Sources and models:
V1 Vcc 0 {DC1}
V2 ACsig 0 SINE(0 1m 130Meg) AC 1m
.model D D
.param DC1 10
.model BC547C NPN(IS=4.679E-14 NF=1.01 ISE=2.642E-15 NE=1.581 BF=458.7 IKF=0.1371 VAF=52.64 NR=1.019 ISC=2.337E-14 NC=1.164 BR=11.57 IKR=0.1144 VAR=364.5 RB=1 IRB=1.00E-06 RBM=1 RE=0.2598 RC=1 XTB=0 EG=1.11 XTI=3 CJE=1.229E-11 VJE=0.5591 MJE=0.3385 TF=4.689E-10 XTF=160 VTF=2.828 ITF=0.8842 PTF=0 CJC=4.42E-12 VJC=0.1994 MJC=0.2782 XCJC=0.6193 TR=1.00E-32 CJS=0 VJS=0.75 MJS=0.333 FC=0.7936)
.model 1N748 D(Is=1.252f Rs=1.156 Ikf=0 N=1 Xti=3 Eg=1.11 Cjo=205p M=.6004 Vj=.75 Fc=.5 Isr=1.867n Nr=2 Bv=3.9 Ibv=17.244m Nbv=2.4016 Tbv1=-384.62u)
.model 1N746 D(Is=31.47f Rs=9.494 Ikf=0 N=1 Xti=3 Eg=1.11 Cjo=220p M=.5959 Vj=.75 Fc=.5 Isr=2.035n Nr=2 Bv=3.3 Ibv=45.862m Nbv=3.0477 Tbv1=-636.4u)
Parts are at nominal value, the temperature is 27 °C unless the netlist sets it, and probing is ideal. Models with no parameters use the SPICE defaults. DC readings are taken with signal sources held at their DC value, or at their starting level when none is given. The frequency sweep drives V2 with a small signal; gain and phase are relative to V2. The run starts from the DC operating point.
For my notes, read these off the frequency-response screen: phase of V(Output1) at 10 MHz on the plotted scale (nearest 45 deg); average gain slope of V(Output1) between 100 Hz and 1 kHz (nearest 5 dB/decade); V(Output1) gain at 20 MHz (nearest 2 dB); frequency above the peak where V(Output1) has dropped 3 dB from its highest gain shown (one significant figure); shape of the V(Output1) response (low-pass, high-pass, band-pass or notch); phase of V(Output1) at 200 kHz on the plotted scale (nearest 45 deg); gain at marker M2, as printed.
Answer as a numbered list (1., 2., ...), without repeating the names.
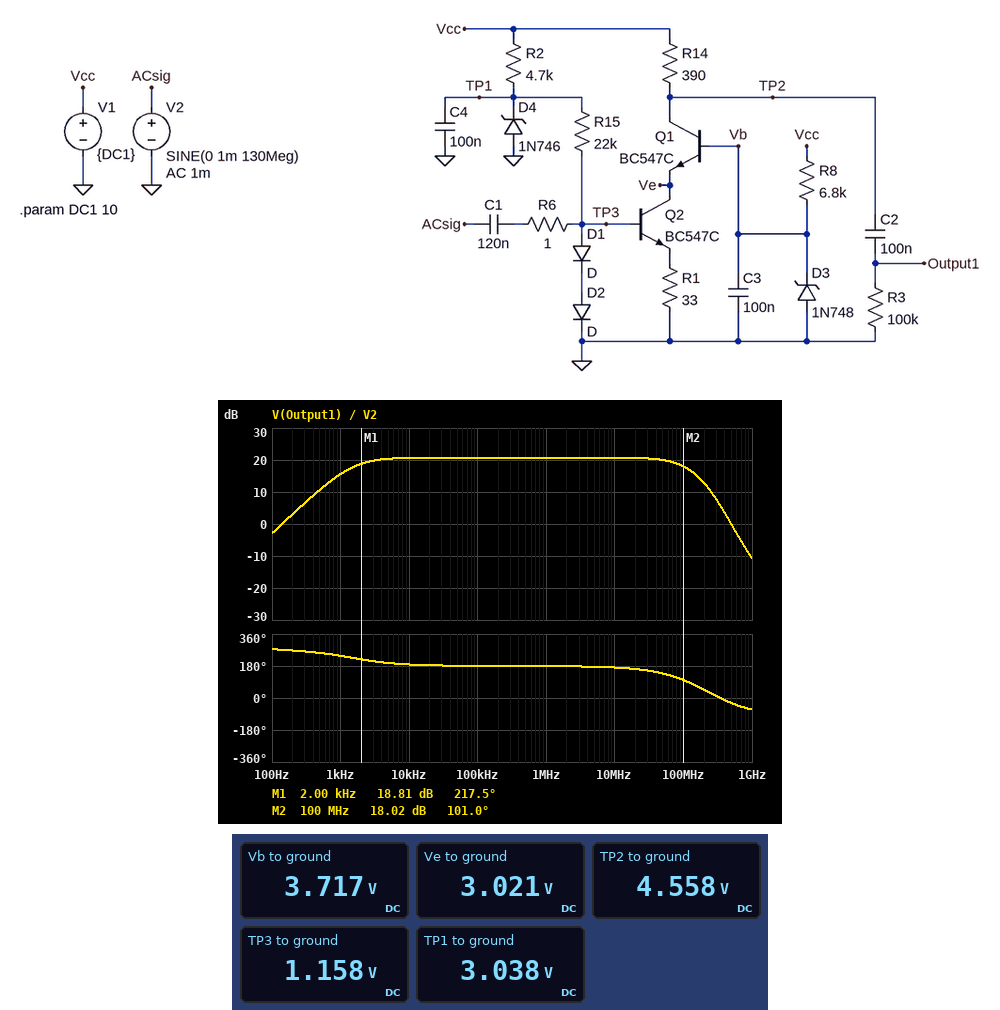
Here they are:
1. 180 deg
2. 20 dB/decade
3. 20 dB
4. 100 MHz
5. band-pass
6. 180 deg
7. 18.02 dB
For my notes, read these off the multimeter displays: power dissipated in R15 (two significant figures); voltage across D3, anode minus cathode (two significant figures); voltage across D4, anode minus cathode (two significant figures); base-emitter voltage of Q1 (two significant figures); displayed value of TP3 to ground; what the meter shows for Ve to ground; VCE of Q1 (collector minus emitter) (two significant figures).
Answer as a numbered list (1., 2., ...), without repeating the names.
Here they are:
1. 160 µW
2. -3.7 V
3. -3.0 V
4. 700 mV
5. 1.158 V
6. 3.021 V
7. 1.5 V
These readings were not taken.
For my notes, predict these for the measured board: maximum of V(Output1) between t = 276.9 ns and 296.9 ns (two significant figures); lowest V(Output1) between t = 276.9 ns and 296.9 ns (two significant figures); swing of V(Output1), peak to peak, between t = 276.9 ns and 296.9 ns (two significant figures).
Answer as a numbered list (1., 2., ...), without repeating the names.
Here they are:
1. 6.7 mV
2. -6.7 mV
3. 13 mV
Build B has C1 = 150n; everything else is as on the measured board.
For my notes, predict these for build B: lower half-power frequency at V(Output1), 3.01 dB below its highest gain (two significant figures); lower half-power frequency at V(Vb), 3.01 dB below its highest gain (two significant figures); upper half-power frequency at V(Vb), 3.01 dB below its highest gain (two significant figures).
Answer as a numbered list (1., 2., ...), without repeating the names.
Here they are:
1. 1.2 kHz
2. 1.1 kHz
3. 25 kHz
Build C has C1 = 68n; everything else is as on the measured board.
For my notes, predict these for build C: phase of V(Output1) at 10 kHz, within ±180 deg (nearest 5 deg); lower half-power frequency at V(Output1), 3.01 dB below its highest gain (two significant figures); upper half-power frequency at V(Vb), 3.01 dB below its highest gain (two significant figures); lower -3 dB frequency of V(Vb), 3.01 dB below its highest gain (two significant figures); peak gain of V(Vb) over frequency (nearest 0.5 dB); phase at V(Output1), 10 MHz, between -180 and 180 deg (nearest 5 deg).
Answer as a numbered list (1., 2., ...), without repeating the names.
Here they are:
1. -165 deg
2. 2.7 kHz
3. 28 kHz
4. 2.2 kHz
5. -46.0 dB
6. 170 deg
